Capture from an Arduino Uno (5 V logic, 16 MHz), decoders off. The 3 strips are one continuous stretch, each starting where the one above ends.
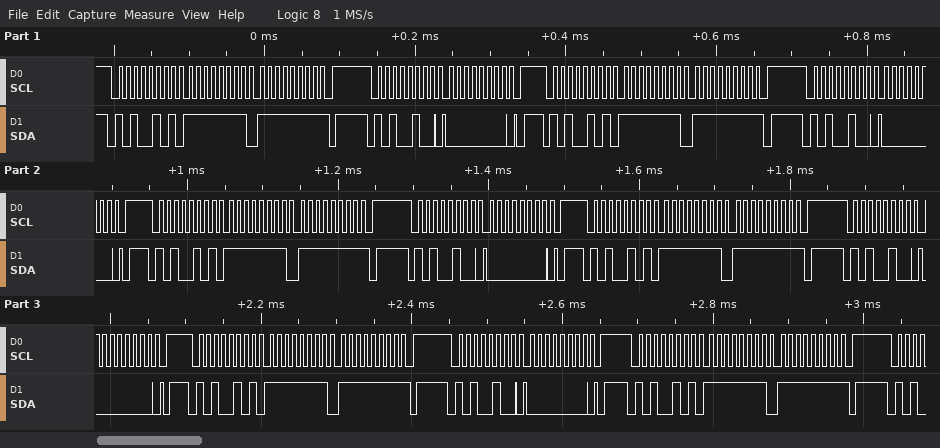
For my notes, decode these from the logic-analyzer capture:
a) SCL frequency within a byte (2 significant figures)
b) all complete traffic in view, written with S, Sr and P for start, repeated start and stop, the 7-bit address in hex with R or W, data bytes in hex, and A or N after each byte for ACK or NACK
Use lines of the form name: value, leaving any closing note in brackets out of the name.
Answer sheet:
SCL frequency within a byte: 100 kHz
all complete traffic in view, written with S, Sr and P for start, repeated start and stop, the 7-bit address in hex with R or W, data bytes in hex, and A or N after each byte for ACK or NACK: S 52R A FF A FF N P S 52W A 00 A P S 52R A FF A FF N P S 52W A 00 A P S 52R A FF A FF N P S 52W A 00 A P S 52R A FF A FF N P S 52W A 00 A P S 52R A FF A FF N P S 52W A 00 A P S 52R A FF A FF N P
